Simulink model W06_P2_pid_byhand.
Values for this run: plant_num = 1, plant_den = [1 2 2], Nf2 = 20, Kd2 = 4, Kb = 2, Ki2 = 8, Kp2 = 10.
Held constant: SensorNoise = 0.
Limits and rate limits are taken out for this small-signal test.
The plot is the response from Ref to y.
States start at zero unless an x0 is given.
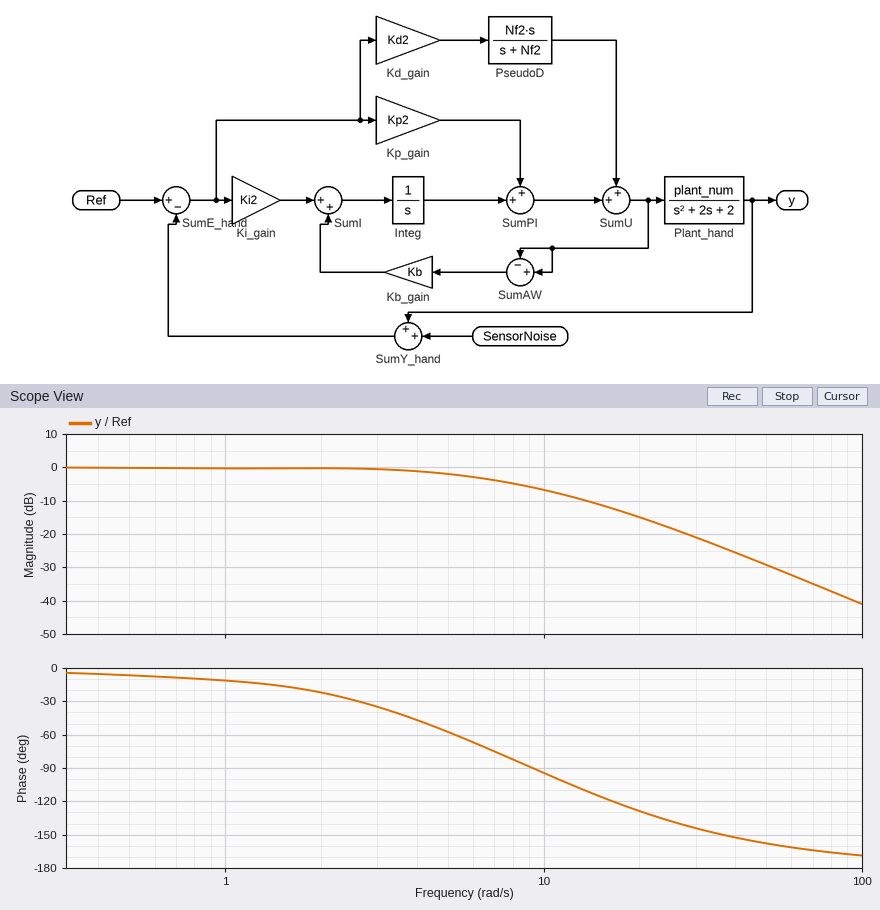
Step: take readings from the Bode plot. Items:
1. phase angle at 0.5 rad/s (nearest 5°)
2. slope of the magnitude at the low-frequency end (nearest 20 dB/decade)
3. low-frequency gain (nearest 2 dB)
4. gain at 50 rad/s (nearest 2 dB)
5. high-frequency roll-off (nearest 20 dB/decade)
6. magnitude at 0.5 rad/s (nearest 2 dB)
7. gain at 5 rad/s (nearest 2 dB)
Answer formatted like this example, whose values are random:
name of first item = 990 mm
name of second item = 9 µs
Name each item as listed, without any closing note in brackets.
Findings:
phase angle at 0.5 rad/s = -5°
slope of the magnitude at the low-frequency end = 0 dB/decade
low-frequency gain = 0 dB
gain at 50 rad/s = -30 dB
high-frequency roll-off = -40 dB/decade
magnitude at 0.5 rad/s = 0 dB
gain at 5 rad/s = -2 dB
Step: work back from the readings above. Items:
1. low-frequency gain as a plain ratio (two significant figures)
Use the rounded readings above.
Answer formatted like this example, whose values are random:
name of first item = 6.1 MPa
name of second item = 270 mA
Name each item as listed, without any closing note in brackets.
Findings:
low-frequency gain as a plain ratio = 1.0
